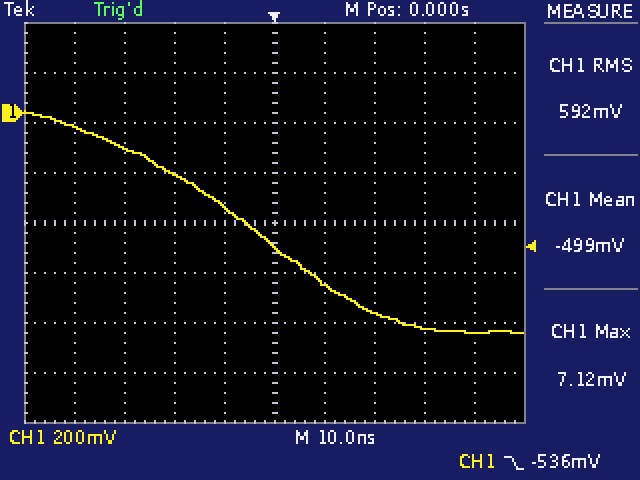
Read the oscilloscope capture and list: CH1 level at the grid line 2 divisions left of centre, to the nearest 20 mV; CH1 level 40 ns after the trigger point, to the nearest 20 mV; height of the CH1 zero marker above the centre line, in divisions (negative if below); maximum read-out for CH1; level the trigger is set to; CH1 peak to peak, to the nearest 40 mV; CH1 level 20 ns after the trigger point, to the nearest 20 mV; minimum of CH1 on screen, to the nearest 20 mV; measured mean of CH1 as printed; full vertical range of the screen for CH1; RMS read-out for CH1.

-240 mV
-880 mV
+2.2 div
7.12 mV
-536 mV
880 mV
-800 mV
-880 mV
-499 mV
1.6 V
592 mV
